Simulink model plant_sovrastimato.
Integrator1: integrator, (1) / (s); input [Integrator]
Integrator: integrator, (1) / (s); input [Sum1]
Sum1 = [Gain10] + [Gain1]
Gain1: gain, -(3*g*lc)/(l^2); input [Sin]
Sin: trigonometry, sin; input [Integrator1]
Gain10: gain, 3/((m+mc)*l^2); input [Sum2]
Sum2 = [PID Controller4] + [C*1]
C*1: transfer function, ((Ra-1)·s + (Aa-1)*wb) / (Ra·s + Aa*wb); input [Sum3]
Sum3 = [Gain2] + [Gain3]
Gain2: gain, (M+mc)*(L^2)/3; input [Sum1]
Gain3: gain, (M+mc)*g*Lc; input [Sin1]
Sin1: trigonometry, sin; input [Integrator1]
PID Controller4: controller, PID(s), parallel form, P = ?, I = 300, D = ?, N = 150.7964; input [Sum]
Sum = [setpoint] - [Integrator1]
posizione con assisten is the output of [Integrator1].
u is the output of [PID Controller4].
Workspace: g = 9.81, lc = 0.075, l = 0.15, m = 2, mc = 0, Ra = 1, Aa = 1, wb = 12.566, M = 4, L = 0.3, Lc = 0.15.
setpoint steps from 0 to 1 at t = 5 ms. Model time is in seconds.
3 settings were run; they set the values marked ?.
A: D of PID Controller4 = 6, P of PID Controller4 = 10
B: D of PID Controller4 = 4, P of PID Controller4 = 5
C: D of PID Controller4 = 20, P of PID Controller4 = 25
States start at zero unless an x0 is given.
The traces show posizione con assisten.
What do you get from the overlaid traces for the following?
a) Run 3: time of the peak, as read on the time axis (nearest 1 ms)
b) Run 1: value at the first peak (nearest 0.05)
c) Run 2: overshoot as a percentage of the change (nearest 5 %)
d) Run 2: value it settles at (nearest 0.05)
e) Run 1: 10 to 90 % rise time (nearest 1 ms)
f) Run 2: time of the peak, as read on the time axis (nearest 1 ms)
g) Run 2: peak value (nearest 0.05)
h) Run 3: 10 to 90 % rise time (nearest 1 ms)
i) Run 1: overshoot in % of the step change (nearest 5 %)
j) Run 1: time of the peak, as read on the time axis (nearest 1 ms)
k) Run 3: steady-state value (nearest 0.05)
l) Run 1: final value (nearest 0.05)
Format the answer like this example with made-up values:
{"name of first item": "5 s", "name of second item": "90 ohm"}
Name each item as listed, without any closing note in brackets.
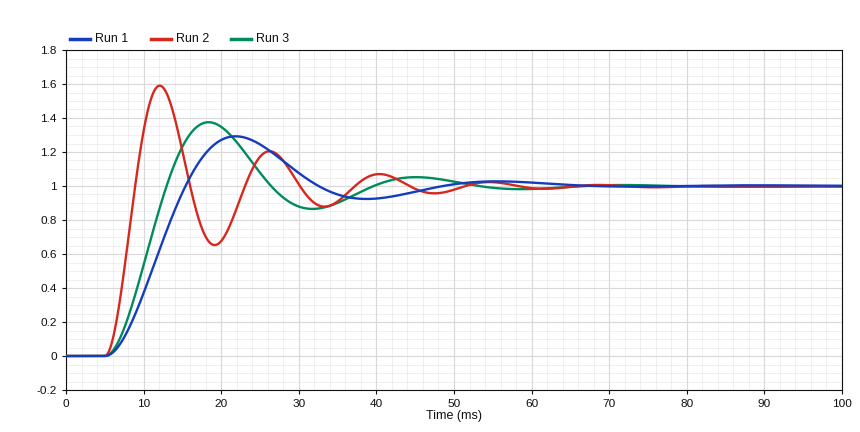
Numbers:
{"Run 3: time of the peak, as read on the time axis": "18 ms", "Run 1: value at the first peak": "1.30", "Run 2: overshoot as a percentage of the change": "60 %", "Run 2: value it settles at": "1.00", "Run 1: 10 to 90 % rise time": "7 ms", "Run 2: time of the peak, as read on the time axis": "12 ms", "Run 2: peak value": "1.60", "Run 3: 10 to 90 % rise time": "5 ms", "Run 1: overshoot in % of the step change": "30 %", "Run 1: time of the peak, as read on the time axis": "22 ms", "Run 3: steady-state value": "1.00", "Run 1: final value": "1.00"}
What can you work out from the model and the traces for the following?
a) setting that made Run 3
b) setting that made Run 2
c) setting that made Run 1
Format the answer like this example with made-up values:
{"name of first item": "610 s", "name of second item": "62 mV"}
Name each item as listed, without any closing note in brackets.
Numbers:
{"setting that made Run 3": "A", "setting that made Run 2": "C", "setting that made Run 1": "B"}
